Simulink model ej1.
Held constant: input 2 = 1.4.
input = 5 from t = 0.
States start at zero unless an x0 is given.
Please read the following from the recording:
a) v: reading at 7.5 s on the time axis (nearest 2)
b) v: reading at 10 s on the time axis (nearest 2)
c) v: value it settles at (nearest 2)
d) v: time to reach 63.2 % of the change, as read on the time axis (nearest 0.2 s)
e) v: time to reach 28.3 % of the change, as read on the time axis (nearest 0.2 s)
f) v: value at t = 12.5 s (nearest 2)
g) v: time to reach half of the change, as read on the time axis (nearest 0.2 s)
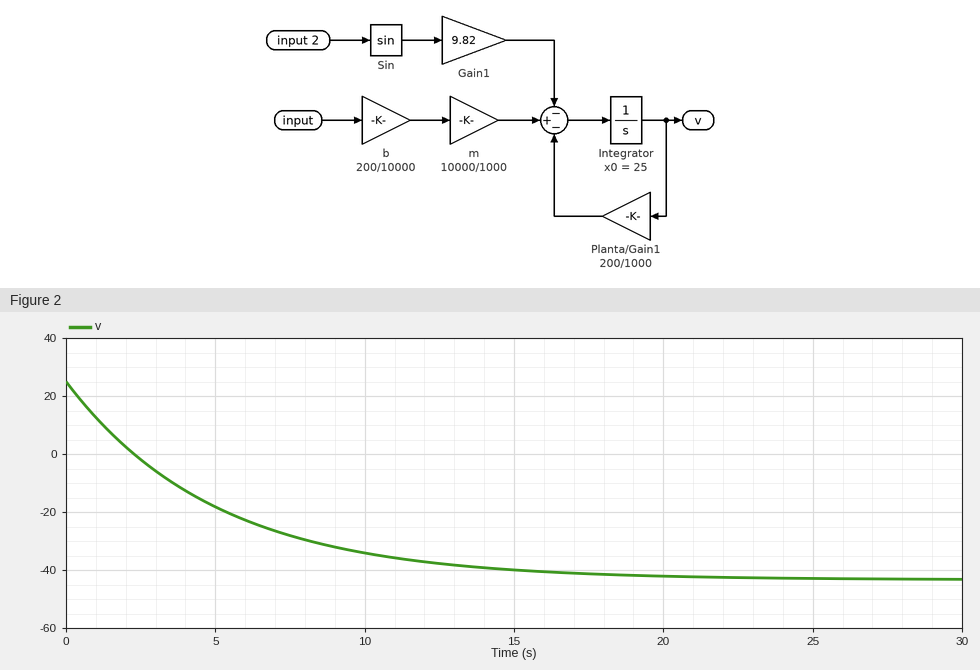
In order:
-28
-34
-44
5.0 s
1.6 s
-38
3.4 s
